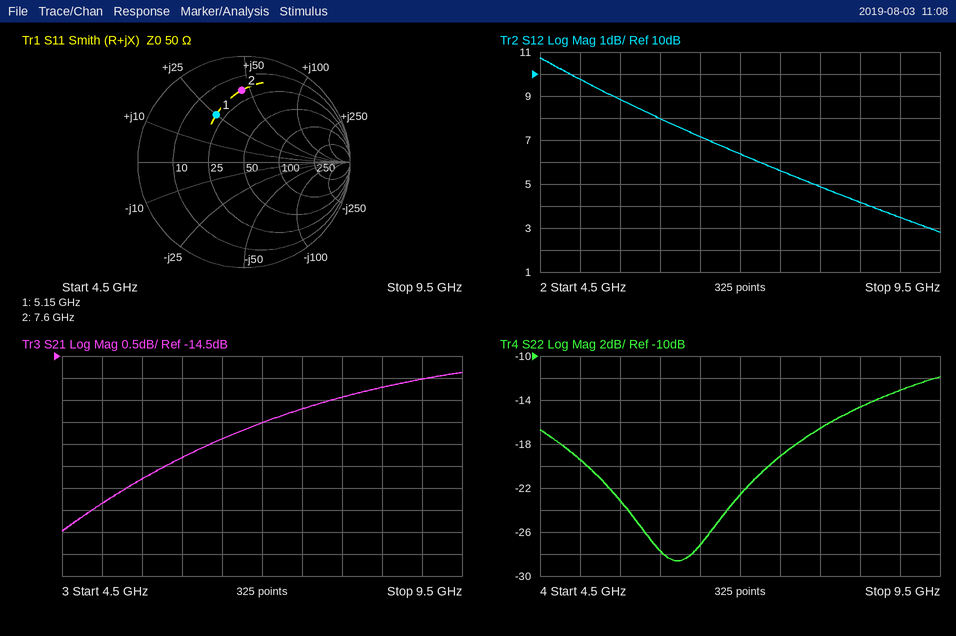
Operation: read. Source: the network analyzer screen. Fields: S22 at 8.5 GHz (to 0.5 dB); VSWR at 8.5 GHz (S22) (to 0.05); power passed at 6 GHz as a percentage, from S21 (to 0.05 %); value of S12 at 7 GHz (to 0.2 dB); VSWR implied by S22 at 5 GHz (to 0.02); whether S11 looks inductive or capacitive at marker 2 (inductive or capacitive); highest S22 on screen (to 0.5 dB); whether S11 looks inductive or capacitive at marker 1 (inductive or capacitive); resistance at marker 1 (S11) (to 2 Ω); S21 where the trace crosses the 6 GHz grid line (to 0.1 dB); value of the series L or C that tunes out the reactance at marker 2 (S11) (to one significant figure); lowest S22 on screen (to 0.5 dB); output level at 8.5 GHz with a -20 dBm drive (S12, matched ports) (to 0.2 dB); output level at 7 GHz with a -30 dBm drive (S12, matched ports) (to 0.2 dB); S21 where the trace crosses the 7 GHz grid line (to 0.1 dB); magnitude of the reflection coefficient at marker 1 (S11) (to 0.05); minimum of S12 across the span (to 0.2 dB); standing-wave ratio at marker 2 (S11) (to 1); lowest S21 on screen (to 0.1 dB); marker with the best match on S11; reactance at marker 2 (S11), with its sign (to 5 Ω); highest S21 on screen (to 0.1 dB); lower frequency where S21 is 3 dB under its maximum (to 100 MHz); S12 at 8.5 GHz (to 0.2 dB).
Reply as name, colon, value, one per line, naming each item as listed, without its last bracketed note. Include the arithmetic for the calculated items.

S22 at 8.5 GHz: -14.5 dB
VSWR at 8.5 GHz (S22): |Γ| = 10^(-14.5/20) = 0.1884; VSWR = (1 + 0.1884)/(1 − 0.1884) ≈ 1.46, so 1.45 to the nearest 0.05
power passed at 6 GHz as a percentage, from S21: 10^(-16.8/10) ≈ 2.09 %, so 2.10 % to the nearest 0.05 %
value of S12 at 7 GHz: 6.4 dB
VSWR implied by S22 at 5 GHz: |Γ| = 10^(-19.5/20) = 0.1059; VSWR = (1 + 0.1059)/(1 − 0.1059) ≈ 1.24
whether S11 looks inductive or capacitive at marker 2: inductive
highest S22 on screen: -12.0 dB
whether S11 looks inductive or capacitive at marker 1: inductive
resistance at marker 1 (S11): 20 Ω
S21 where the trace crosses the 6 GHz grid line: -16.8 dB
value of the series L or C that tunes out the reactance at marker 2 (S11): C = 1/(2π × 7.6 GHz × 45 Ω) ≈ 465 fF, so 500 fF to one significant figure
lowest S22 on screen: -28.5 dB
output level at 8.5 GHz with a -20 dBm drive (S12, matched ports): -20 dBm + (4.2 dB) = -15.8 dBm
output level at 7 GHz with a -30 dBm drive (S12, matched ports): -30 dBm + (6.4 dB) = -23.6 dBm
S21 where the trace crosses the 7 GHz grid line: -16.0 dB
magnitude of the reflection coefficient at marker 1 (S11): 0.50
minimum of S12 across the span: 2.8 dB
standing-wave ratio at marker 2 (S11): 5
lowest S21 on screen: -18.5 dB
marker with the best match on S11: marker 1
reactance at marker 2 (S11), with its sign: +45 Ω
highest S21 on screen: -14.9 dB
lower frequency where S21 is 3 dB under its maximum: 5.0 GHz
S12 at 8.5 GHz: 4.2 dB
